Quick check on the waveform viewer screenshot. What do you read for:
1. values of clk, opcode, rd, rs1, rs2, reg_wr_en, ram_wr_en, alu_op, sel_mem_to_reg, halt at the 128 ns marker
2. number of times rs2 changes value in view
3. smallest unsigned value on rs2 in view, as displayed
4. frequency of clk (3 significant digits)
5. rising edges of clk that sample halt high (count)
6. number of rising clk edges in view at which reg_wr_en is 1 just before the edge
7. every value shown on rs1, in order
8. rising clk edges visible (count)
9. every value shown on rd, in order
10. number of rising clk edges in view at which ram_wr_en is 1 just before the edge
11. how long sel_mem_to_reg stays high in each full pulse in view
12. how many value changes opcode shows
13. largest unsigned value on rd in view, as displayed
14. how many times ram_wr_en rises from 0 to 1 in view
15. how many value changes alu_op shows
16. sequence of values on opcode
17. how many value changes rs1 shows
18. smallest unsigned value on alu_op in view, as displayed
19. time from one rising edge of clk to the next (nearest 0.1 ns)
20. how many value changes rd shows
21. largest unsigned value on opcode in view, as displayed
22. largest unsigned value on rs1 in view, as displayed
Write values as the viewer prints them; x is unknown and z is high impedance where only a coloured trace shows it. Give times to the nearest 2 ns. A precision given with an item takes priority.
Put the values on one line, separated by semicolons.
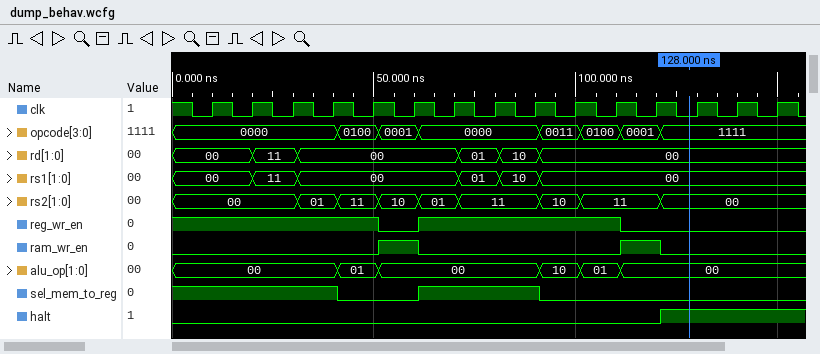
clk=0, opcode=1111, rd=00, rs1=00, rs2=00, reg_wr_en=0, ram_wr_en=0, alu_op=00, sel_mem_to_reg=0, halt=1; 8; 00; 100 MHz; 3; 10; 00, 11, 00, 01, 10, 00; 15; 00, 11, 00, 01, 10, 00; 2; 30 ns; 7; 11; 2; 5; 0000, 0100, 0001, 0000, 0011, 0100, 0001, 1111; 5; 00; 10 ns; 5; 1111; 11
